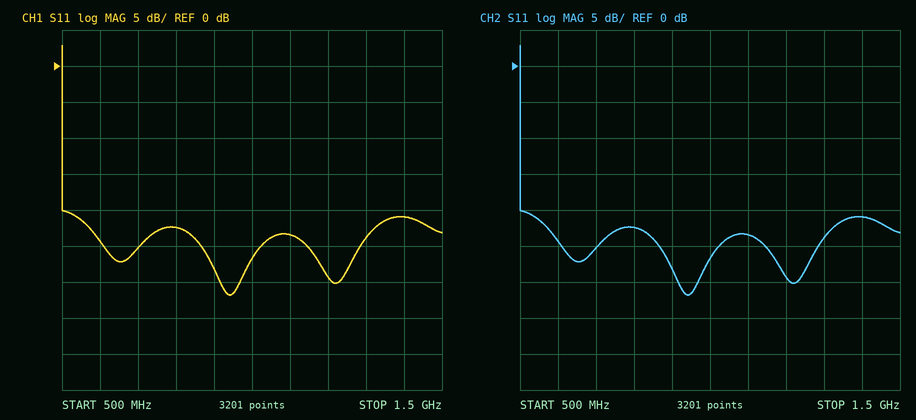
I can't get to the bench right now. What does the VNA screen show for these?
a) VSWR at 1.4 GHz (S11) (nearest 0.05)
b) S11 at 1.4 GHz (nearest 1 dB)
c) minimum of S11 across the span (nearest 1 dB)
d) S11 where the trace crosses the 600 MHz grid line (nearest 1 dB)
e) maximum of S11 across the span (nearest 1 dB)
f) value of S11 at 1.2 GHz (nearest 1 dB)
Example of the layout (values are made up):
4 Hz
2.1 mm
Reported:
1.20
-21 dB
-32 dB
-24 dB
3 dB
-29 dB
